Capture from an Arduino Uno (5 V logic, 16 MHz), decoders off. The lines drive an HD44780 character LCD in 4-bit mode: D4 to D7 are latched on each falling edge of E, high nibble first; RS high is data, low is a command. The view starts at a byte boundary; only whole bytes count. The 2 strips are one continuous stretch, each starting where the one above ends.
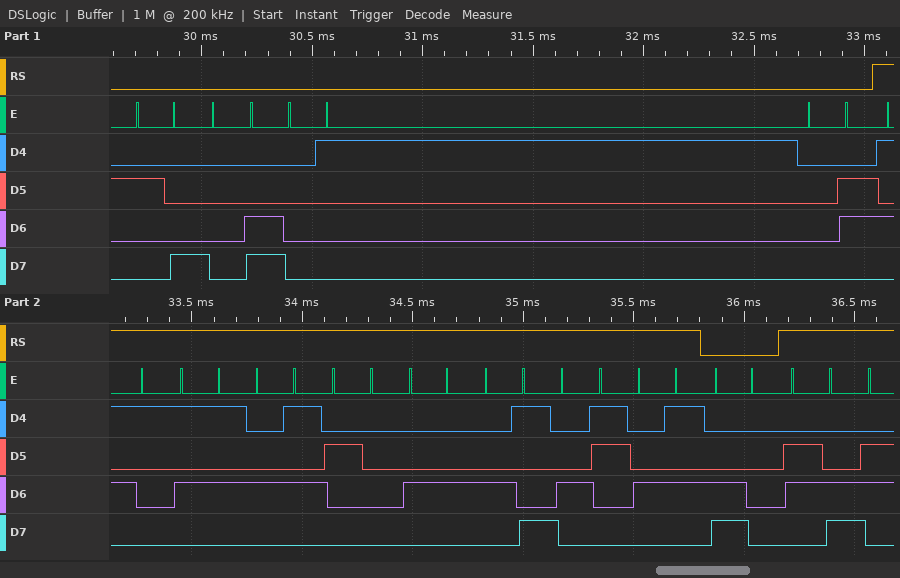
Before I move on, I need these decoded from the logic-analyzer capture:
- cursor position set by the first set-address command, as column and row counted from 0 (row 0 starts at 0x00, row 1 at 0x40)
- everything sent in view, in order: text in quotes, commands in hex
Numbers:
column 0, row 1
0x28 0x0C 0x01 0x06 "QUE DICE" 0xC0 "l"
